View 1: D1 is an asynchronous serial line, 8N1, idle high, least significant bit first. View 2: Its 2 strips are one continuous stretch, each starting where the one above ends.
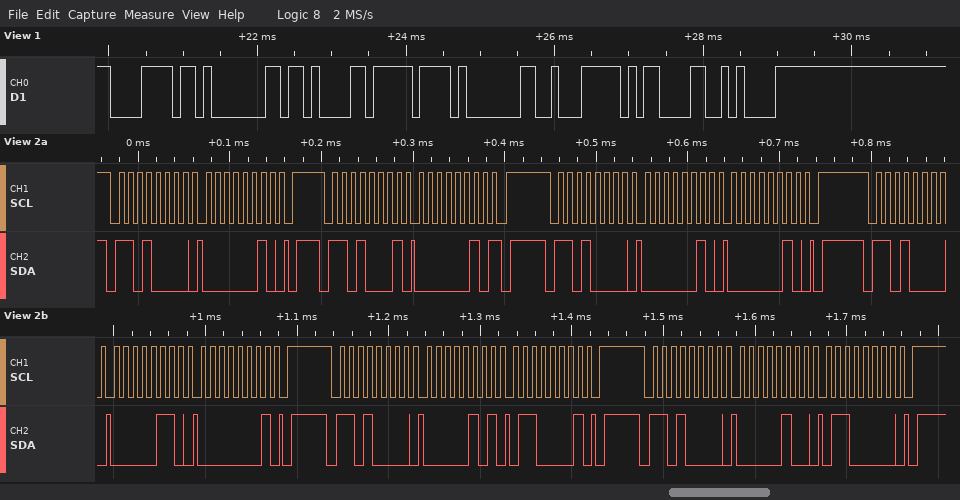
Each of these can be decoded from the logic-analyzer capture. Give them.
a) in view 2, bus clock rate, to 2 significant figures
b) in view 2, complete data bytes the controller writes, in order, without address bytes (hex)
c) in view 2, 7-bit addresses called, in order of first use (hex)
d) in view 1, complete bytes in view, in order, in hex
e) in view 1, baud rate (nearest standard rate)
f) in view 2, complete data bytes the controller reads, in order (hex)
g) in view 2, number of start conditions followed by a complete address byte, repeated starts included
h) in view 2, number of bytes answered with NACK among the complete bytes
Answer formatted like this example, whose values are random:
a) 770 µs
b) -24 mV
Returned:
a) 100 kHz
b) 02 02 02 06 01 05 61 04 60
c) 0x68
d) 78 01 0B DF 01 E2 0D 0A
e) 9600 baud
f) 02
g) 6
h) 1
